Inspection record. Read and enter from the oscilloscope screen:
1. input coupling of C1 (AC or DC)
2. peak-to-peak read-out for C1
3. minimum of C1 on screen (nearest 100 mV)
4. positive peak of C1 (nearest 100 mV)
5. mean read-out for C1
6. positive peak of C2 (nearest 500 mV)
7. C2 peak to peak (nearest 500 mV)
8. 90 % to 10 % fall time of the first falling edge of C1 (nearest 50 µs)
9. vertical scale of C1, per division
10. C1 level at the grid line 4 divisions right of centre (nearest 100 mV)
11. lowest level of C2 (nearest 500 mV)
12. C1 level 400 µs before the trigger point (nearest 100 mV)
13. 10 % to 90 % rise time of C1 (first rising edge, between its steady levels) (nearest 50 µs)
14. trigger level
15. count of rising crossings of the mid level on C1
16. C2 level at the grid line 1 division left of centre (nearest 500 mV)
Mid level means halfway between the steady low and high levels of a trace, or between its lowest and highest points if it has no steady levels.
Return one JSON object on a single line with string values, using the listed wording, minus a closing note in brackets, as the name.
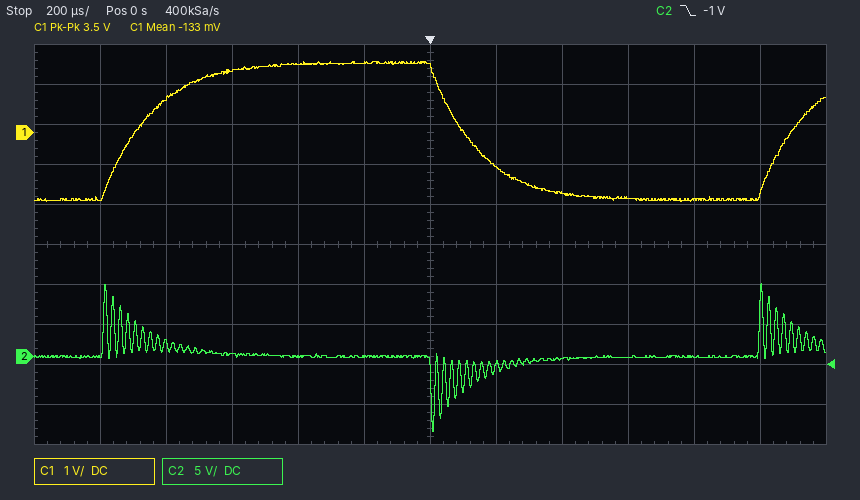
{"input coupling of C1": "DC", "peak-to-peak read-out for C1": "3.5 V", "minimum of C1 on screen": "-1.7 V", "positive peak of C1": "1.8 V", "mean read-out for C1": "-133 mV", "positive peak of C2": "9.0 V", "C2 peak to peak": "18.5 V", "90 % to 10 % fall time of the first falling edge of C1": "300 µs", "vertical scale of C1, per division": "1 V", "C1 level at the grid line 4 divisions right of centre": "-1.7 V", "lowest level of C2": "-9.5 V", "C1 level 400 µs before the trigger point": "1.7 V", "10 % to 90 % rise time of C1 (first rising edge, between its steady levels)": "300 µs", "trigger level": "-1 V", "count of rising crossings of the mid level on C1": "2", "C2 level at the grid line 1 division left of centre": "0.0 V"}
